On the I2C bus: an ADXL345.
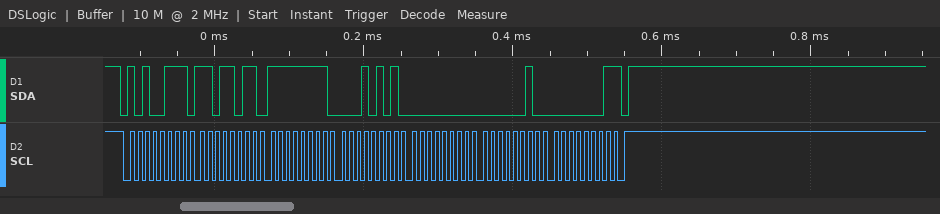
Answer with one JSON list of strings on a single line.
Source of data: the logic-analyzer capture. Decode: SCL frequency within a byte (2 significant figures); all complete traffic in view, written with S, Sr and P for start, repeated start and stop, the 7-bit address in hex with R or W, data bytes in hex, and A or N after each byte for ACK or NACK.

["100 kHz", "S 53R A DB A FF A 15 A 00 A 02 A 01 N P"]
